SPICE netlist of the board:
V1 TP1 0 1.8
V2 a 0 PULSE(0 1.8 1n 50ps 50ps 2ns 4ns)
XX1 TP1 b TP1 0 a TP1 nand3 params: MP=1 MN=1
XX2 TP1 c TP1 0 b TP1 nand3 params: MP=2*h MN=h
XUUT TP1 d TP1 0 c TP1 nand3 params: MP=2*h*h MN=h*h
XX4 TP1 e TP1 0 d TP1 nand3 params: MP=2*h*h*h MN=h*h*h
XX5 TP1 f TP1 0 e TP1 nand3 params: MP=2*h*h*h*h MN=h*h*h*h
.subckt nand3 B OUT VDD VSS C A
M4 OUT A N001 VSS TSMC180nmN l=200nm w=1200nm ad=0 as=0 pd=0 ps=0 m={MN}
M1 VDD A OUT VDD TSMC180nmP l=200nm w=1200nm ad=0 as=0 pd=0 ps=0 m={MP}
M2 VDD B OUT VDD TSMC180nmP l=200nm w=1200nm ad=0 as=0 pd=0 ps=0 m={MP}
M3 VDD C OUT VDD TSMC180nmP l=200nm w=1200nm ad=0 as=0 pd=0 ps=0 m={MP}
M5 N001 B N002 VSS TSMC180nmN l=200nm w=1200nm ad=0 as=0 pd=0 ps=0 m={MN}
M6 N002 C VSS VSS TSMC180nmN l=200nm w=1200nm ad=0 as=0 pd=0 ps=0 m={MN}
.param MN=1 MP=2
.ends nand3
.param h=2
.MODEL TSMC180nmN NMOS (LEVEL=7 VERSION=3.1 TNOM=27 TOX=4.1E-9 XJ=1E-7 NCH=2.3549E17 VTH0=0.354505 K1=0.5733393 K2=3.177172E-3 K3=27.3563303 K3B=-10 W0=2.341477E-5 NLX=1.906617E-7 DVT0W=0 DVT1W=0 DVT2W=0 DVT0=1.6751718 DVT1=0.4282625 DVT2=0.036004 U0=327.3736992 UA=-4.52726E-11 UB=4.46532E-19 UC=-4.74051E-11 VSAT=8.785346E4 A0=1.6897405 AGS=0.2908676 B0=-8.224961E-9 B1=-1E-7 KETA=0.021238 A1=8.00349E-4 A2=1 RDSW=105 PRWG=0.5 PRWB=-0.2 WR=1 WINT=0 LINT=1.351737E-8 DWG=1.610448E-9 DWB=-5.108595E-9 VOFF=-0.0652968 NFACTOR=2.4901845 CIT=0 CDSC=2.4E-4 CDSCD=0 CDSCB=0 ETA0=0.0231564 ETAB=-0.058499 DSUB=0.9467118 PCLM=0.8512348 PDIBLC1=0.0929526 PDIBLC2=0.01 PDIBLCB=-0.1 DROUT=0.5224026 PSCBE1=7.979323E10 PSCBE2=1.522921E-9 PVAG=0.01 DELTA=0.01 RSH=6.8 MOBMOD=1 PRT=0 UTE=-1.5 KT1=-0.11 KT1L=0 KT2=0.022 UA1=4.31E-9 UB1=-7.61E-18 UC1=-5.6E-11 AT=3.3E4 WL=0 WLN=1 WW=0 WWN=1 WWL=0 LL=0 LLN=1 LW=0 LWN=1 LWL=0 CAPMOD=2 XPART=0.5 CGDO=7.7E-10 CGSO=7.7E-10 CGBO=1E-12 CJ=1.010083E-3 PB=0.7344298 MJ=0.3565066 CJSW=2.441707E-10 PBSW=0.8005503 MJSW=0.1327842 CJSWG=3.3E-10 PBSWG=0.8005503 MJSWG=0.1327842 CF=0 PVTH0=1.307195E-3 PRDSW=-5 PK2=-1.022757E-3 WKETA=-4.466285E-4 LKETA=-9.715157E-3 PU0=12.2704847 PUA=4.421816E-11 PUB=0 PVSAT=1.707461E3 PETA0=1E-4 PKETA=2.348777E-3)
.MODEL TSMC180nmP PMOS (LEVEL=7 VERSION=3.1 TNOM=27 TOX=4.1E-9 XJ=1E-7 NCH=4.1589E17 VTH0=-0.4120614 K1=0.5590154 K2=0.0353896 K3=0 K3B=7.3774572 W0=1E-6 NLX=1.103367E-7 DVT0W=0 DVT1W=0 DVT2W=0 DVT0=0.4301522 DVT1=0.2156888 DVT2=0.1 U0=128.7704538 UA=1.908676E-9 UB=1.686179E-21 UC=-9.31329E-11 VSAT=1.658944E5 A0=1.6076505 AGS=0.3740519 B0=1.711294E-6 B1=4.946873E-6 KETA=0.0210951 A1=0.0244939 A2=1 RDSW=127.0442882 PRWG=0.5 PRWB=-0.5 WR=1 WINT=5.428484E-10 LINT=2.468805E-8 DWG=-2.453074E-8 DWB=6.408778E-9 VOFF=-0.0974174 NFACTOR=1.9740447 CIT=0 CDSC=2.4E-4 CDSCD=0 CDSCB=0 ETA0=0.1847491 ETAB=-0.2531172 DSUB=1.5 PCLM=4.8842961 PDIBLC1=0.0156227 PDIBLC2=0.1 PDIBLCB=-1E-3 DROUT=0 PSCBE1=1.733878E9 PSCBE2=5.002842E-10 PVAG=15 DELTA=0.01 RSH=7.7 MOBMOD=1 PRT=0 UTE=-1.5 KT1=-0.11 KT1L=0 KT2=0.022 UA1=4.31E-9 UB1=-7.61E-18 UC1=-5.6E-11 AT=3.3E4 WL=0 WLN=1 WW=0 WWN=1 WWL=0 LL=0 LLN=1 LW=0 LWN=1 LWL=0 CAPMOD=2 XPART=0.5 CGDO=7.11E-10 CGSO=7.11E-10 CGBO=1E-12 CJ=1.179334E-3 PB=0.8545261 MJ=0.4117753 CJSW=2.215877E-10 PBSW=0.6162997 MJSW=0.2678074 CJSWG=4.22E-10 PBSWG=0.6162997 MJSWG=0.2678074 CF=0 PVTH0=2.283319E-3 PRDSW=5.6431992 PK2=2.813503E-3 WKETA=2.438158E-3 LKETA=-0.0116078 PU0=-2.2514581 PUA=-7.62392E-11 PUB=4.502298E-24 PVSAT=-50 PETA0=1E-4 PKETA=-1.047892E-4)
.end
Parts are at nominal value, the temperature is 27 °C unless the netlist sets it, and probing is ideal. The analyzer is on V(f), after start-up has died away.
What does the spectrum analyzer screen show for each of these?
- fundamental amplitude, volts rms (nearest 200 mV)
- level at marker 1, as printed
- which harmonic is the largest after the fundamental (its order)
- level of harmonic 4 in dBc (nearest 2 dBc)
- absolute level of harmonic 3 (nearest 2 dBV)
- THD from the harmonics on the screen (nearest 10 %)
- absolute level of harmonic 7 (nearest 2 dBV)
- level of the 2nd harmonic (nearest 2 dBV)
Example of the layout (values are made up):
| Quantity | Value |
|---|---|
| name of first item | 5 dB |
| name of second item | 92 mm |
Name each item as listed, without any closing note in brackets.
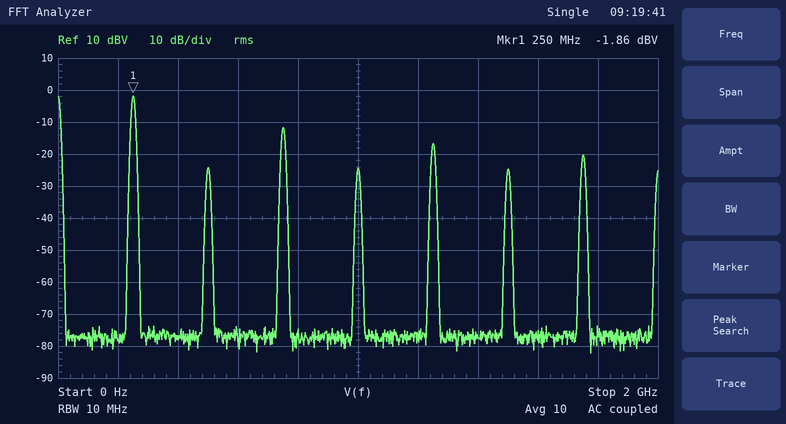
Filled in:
| Quantity | Value |
|---|---|
| fundamental amplitude, volts rms | 800 mV |
| level at marker 1, as printed | -1.86 dBV |
| which harmonic is the largest after the fundamental | 3 |
| level of harmonic 4 in dBc | -22 dBc |
| absolute level of harmonic 3 | -12 dBV |
| THD from the harmonics on the screen | 40 % |
| absolute level of harmonic 7 | -20 dBV |
| level of the 2nd harmonic | -24 dBV |
